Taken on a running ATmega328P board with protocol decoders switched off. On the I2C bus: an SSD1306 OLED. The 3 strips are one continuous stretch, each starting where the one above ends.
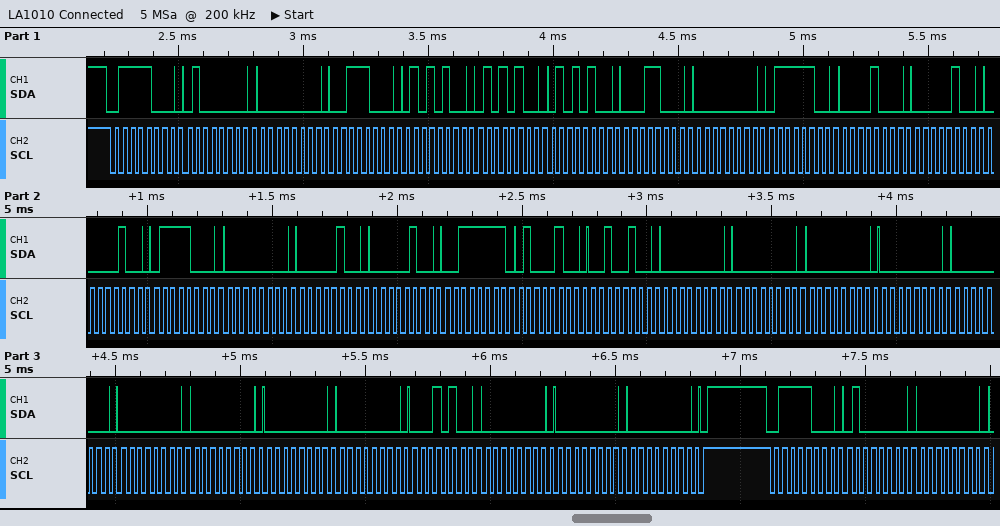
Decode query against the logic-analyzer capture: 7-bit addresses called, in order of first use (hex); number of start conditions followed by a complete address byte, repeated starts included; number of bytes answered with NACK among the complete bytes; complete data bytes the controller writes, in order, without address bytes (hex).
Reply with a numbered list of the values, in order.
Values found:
1. 0x3C
2. 2
3. 0
4. 40 00 38 54 54 54 18 00 7C 08 04 04 78 00 04 04 3F 44 24 00 00 00 00 00 00 00 00 00 14 00 00 00 40 00
